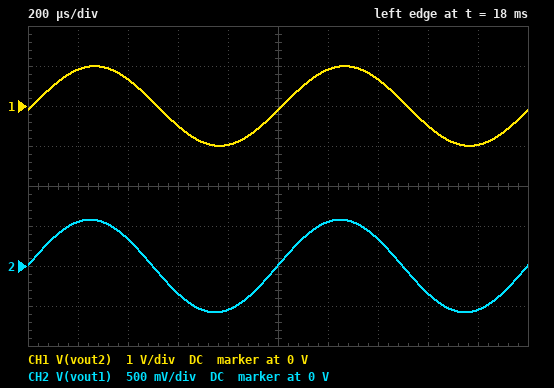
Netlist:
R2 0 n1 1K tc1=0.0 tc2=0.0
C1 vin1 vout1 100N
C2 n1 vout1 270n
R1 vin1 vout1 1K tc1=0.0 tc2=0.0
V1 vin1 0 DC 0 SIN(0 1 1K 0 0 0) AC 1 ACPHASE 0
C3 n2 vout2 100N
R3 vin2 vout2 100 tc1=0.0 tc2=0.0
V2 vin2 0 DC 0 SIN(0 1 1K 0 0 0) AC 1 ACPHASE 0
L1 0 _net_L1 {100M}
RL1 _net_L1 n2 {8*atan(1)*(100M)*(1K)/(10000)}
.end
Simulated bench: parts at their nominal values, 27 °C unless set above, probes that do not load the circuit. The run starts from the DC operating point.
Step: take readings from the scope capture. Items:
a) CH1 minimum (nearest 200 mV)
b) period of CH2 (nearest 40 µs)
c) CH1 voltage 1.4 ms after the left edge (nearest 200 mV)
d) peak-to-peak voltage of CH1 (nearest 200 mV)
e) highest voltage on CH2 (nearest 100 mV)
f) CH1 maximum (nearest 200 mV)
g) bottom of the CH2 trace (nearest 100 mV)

-1.0 V
1.00 ms
600 mV
2.0 V
600 mV
1.0 V
-600 mV
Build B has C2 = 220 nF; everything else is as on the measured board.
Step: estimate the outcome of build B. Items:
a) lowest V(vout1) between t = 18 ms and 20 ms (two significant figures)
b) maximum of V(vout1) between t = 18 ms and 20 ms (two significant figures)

-590 mV
590 mV
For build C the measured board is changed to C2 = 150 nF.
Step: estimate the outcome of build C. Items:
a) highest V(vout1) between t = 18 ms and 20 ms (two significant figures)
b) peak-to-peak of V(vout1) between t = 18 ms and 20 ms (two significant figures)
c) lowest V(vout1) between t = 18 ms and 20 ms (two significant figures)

640 mV
1.3 V
-640 mV
